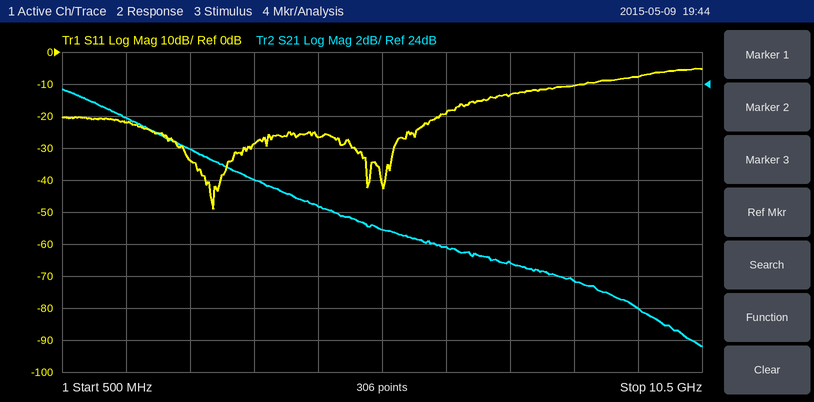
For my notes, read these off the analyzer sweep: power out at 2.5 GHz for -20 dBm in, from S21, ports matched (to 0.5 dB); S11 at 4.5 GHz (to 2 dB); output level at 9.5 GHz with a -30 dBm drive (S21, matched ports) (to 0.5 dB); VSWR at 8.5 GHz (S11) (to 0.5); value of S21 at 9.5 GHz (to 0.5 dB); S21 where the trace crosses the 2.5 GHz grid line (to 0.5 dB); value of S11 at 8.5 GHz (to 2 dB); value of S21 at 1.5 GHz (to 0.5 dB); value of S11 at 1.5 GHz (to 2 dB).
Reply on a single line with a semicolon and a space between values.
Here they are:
0.0 dBm; -26 dB; -20.0 dBm; 2.0; 10.0 dB; 20.0 dB; -10 dB; 22.0 dB; -22 dB
